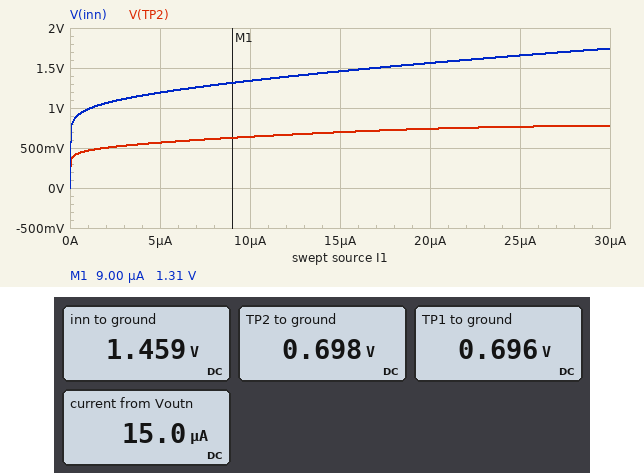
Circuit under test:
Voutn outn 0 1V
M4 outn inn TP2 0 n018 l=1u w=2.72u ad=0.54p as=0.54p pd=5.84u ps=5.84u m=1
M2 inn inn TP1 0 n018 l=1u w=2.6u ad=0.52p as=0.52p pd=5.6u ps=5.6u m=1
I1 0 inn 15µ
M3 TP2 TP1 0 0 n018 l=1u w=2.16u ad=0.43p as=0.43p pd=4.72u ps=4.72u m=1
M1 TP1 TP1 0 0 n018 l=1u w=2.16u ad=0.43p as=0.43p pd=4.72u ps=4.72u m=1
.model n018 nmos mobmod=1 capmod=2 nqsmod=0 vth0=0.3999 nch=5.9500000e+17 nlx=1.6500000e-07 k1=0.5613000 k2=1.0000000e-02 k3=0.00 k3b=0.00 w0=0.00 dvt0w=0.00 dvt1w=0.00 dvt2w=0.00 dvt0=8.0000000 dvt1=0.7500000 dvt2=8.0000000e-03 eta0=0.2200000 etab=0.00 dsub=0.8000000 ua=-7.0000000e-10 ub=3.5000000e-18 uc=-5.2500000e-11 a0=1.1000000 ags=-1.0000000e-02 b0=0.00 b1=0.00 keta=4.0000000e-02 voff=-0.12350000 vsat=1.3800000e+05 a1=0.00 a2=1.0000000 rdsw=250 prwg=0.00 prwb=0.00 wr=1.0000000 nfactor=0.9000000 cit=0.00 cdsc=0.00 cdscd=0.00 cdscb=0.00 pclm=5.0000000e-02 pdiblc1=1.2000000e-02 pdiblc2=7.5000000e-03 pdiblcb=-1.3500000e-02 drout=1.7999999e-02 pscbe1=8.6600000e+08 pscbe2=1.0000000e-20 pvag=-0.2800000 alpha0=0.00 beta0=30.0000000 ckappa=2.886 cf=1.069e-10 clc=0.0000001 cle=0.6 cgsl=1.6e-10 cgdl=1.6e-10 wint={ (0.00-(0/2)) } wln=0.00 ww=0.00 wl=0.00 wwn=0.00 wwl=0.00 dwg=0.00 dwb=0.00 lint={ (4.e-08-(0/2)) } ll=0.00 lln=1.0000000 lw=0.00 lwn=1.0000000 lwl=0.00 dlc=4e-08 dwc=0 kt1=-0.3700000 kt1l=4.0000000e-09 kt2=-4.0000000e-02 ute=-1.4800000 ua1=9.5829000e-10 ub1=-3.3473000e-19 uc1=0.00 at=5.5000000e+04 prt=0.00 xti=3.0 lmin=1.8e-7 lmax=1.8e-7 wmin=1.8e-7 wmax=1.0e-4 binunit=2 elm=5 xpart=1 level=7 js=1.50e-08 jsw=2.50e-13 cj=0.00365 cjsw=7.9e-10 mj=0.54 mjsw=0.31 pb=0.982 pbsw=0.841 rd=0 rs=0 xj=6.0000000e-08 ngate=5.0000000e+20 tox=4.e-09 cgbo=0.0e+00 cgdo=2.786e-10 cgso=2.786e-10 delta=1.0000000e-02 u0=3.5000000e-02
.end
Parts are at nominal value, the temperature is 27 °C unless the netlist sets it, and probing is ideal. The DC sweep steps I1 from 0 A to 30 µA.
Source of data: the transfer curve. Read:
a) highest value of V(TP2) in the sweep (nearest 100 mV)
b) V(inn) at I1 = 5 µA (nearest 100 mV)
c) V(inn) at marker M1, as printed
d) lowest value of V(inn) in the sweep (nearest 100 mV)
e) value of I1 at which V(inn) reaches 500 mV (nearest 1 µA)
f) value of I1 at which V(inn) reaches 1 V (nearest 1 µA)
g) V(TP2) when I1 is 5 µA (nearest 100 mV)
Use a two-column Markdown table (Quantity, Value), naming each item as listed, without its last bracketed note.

| Quantity | Value |
|---|---|
| highest value of V(TP2) in the sweep | 800 mV |
| V(inn) at I1 = 5 µA | 1.2 V |
| V(inn) at marker M1, as printed | 1.31 V |
| lowest value of V(inn) in the sweep | 0 V |
| value of I1 at which V(inn) reaches 500 mV | 0 A |
| value of I1 at which V(inn) reaches 1 V | 1 µA |
| V(TP2) when I1 is 5 µA | 600 mV |
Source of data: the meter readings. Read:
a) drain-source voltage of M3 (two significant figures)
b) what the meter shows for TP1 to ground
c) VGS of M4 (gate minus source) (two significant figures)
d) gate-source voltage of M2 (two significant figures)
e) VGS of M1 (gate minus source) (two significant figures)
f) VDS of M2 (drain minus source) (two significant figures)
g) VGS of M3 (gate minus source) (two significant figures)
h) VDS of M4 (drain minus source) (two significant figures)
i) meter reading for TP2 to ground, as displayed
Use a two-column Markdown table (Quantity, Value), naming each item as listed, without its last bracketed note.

| Quantity | Value |
|---|---|
| drain-source voltage of M3 | 700 mV |
| what the meter shows for TP1 to ground | 0.696 V |
| VGS of M4 (gate minus source) | 760 mV |
| gate-source voltage of M2 | 760 mV |
| VGS of M1 (gate minus source) | 700 mV |
| VDS of M2 (drain minus source) | 760 mV |
| VGS of M3 (gate minus source) | 700 mV |
| VDS of M4 (drain minus source) | 300 mV |
| meter reading for TP2 to ground, as displayed | 0.698 V |
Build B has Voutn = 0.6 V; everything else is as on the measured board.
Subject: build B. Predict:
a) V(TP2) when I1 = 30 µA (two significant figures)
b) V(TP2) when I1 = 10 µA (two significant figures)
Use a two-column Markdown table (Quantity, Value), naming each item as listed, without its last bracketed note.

| Quantity | Value |
|---|---|
| V(TP2) when I1 = 30 µA | 490 mV |
| V(TP2) when I1 = 10 µA | 520 mV |
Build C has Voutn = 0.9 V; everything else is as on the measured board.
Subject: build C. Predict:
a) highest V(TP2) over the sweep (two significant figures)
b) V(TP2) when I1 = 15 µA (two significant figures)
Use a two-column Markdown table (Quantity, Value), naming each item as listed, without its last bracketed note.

| Quantity | Value |
|---|---|
| highest V(TP2) over the sweep | 720 mV |
| V(TP2) when I1 = 15 µA | 690 mV |
